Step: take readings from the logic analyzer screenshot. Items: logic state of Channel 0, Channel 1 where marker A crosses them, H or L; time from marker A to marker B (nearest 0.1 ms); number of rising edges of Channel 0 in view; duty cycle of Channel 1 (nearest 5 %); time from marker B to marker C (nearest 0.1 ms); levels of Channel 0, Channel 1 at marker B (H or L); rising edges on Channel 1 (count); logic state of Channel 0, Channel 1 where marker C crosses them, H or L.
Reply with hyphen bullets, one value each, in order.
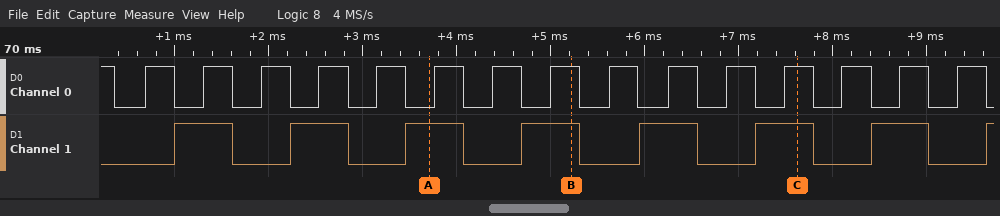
- Channel 0=L, Channel 1=H
- 1.5 ms
- 15
- 50 %
- 2.4 ms
- Channel 0=H, Channel 1=H
- 8
- Channel 0=H, Channel 1=H
